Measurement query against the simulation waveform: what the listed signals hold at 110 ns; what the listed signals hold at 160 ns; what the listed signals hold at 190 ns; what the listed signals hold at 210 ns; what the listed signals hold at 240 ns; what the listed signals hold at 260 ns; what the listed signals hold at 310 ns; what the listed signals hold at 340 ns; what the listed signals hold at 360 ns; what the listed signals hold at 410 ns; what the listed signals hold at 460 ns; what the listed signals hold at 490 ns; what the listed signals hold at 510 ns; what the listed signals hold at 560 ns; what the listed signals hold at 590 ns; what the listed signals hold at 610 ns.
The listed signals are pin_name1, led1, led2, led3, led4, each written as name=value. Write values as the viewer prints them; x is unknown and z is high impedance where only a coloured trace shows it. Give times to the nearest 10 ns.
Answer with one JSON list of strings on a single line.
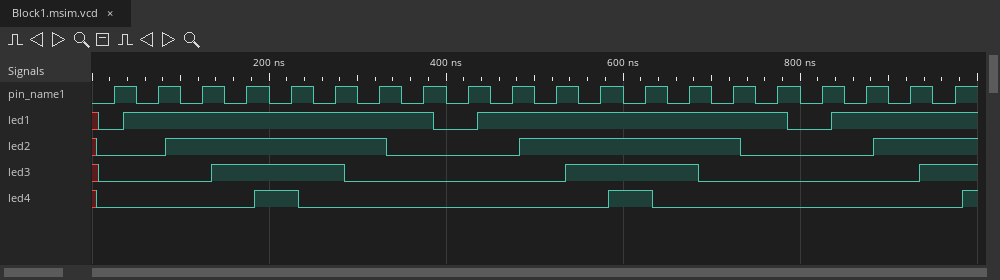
["pin_name1=0, led1=1, led2=1, led3=0, led4=0", "pin_name1=0, led1=1, led2=1, led3=1, led4=0", "pin_name1=1, led1=1, led2=1, led3=1, led4=1", "pin_name1=0, led1=1, led2=1, led3=1, led4=1", "pin_name1=1, led1=1, led2=1, led3=1, led4=0", "pin_name1=0, led1=1, led2=1, led3=1, led4=0", "pin_name1=0, led1=1, led2=1, led3=0, led4=0", "pin_name1=1, led1=1, led2=0, led3=0, led4=0", "pin_name1=0, led1=1, led2=0, led3=0, led4=0", "pin_name1=0, led1=0, led2=0, led3=0, led4=0", "pin_name1=0, led1=1, led2=0, led3=0, led4=0", "pin_name1=1, led1=1, led2=1, led3=0, led4=0", "pin_name1=0, led1=1, led2=1, led3=0, led4=0", "pin_name1=0, led1=1, led2=1, led3=1, led4=0", "pin_name1=1, led1=1, led2=1, led3=1, led4=1", "pin_name1=0, led1=1, led2=1, led3=1, led4=1"]
